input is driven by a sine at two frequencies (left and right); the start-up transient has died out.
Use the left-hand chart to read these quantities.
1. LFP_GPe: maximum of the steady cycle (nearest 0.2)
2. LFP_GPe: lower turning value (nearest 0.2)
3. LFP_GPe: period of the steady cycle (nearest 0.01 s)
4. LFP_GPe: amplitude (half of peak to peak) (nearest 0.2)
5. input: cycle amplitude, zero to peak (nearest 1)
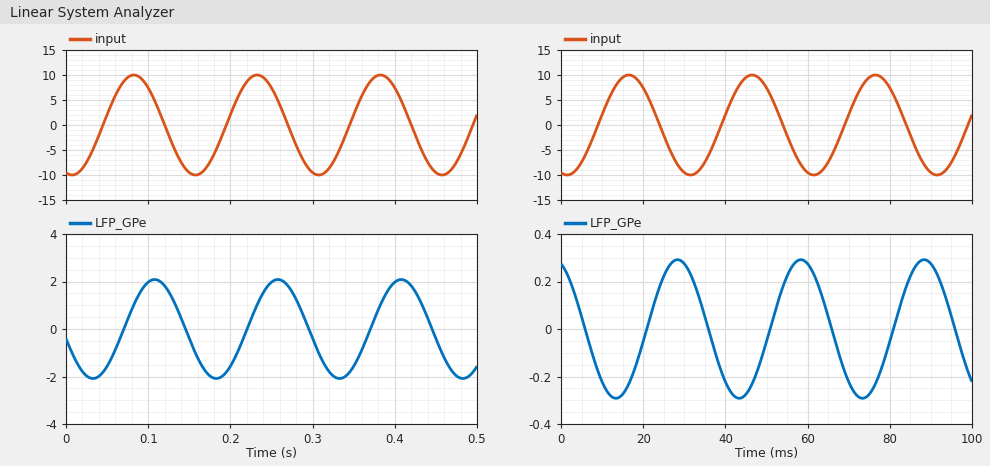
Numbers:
2.0
-2.0
0.15 s
2.0
10
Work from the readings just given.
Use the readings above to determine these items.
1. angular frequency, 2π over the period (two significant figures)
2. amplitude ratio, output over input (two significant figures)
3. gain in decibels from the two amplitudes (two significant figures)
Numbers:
42 rad/s
0.20
-14 dB
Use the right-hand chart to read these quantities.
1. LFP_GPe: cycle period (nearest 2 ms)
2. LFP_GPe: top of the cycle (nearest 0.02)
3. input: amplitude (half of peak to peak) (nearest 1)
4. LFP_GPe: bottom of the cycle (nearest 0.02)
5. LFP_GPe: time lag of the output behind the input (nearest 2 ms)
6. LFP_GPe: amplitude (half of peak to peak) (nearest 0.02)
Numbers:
30 ms
0.30
10
-0.30
12 ms
0.30
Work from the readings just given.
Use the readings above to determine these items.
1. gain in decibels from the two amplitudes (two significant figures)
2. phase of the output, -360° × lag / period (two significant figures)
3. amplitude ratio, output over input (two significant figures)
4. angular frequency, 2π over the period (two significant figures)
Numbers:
-30 dB
-140°
0.030
0.21 rad/ms
